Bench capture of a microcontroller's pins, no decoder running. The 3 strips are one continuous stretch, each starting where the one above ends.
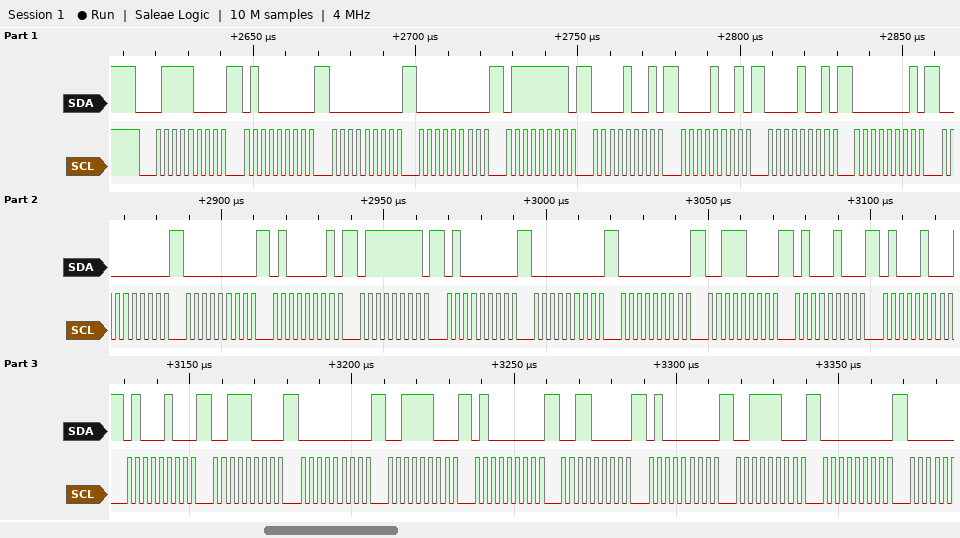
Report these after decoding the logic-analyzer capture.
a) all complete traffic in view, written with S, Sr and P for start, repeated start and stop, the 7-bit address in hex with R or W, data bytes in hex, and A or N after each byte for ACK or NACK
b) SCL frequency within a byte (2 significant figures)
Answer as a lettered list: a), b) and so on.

a) S 3CW A 40 A 00 A 00 A 7F A 09 A 09 A 09 A 01 A 00 A 00 A 41 A 7F A 40 A 00 A 00 A 38 A 44 A 44 A 44 A 38 A 00 A 3C A 40 A 30 A 40 A 3C A 00 A
b) 400 kHz
